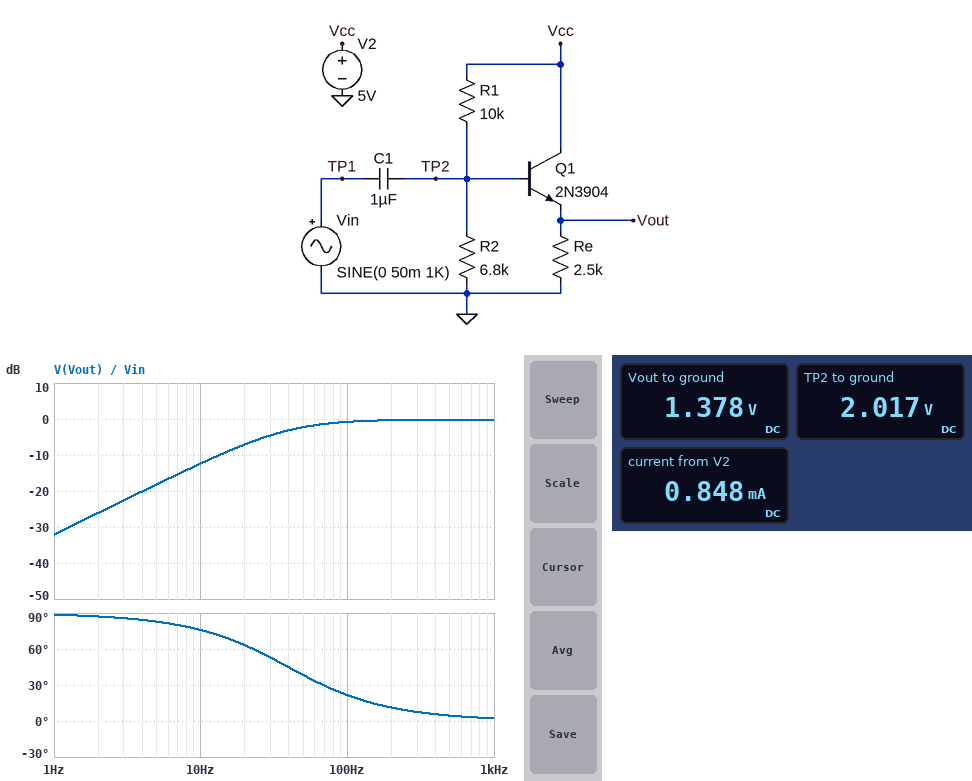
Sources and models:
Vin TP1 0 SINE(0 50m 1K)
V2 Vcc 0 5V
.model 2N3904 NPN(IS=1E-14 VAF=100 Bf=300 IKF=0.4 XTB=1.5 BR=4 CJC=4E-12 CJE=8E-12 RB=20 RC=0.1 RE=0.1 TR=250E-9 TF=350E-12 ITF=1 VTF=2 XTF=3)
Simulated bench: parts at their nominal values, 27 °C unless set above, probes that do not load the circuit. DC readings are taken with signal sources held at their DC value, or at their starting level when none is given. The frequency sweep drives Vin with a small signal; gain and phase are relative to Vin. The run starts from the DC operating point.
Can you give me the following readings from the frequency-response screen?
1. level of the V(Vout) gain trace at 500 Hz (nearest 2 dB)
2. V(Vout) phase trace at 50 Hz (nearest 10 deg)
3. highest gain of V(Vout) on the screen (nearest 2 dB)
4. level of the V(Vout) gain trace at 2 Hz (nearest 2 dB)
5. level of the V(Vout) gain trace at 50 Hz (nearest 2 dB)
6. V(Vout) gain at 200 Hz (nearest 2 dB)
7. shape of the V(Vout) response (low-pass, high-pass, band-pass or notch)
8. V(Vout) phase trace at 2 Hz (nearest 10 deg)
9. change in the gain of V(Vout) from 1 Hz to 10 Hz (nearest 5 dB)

0 dB
40 deg
0 dB
-26 dB
-2 dB
0 dB
high-pass
90 deg
20 dB
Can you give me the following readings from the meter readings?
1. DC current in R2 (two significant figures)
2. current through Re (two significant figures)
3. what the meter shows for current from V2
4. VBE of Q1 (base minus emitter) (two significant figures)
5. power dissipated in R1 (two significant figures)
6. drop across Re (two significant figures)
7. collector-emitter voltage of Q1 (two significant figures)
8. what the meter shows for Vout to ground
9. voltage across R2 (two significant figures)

300 µA
550 µA
0.848 mA
640 mV
890 µW
1.4 V
3.6 V
1.378 V
2.0 V
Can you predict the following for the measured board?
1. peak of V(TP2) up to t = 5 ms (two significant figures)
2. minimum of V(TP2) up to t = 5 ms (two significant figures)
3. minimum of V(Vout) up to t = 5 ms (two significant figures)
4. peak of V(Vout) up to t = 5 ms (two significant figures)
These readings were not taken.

2.1 V
2.0 V
1.3 V
1.4 V
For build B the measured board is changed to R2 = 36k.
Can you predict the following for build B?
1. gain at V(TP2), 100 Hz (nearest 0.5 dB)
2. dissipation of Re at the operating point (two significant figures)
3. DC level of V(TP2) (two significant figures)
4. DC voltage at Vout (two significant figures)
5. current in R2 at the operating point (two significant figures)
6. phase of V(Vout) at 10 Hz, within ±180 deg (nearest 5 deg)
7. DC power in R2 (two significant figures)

0 dB
4.1 mW
3.9 V
3.2 V
110 µA
65 deg
420 µW
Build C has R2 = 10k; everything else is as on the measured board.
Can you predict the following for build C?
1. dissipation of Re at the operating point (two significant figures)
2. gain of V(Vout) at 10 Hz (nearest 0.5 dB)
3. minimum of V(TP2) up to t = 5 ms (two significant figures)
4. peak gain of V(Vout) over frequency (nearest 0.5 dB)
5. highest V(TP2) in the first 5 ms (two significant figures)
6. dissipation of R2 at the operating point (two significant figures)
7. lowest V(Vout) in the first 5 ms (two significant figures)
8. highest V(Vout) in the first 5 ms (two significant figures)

1.4 mW
-10.5 dB
2.4 V
0 dB
2.5 V
620 µW
1.8 V
1.9 V
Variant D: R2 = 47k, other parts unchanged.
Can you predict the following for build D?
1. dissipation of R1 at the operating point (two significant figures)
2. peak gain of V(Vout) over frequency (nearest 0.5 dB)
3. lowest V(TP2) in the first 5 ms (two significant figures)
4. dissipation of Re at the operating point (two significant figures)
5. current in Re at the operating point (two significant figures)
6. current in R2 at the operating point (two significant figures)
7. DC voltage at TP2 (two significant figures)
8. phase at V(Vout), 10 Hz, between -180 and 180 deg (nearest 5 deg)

84 µW
0 dB
4.0 V
4.7 mW
1.4 mA
87 µA
4.1 V
65 deg
